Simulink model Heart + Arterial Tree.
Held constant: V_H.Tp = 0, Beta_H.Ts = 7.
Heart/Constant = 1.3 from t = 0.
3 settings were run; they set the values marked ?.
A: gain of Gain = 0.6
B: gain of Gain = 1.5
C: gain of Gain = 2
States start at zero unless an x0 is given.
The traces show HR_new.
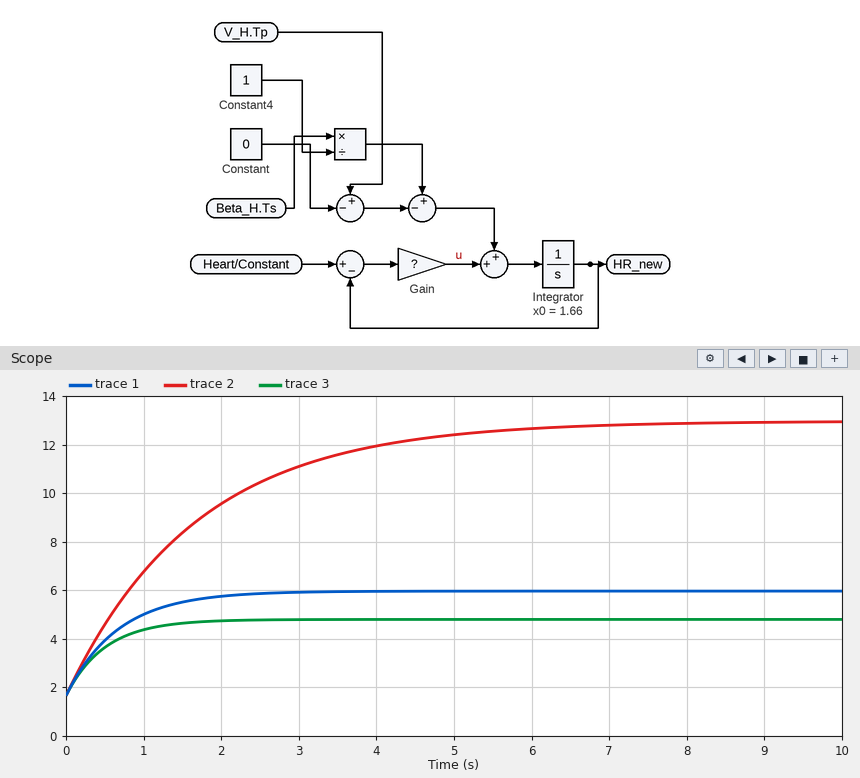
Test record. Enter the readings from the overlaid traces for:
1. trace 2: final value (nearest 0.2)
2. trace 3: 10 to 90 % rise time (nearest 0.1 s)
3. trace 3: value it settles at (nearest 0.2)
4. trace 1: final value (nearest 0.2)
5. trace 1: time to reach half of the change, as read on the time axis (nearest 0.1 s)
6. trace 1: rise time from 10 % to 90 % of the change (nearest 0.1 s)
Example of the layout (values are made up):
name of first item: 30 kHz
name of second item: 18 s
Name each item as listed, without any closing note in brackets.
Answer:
trace 2: final value: 13.0
trace 3: 10 to 90 % rise time: 1.1 s
trace 3: value it settles at: 4.8
trace 1: final value: 6.0
trace 1: time to reach half of the change, as read on the time axis: 0.5 s
trace 1: rise time from 10 % to 90 % of the change: 1.5 s
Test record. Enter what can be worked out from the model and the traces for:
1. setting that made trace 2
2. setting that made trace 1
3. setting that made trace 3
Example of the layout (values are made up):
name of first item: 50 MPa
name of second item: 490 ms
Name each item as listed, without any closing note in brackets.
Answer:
setting that made trace 2: A
setting that made trace 1: B
setting that made trace 3: C
